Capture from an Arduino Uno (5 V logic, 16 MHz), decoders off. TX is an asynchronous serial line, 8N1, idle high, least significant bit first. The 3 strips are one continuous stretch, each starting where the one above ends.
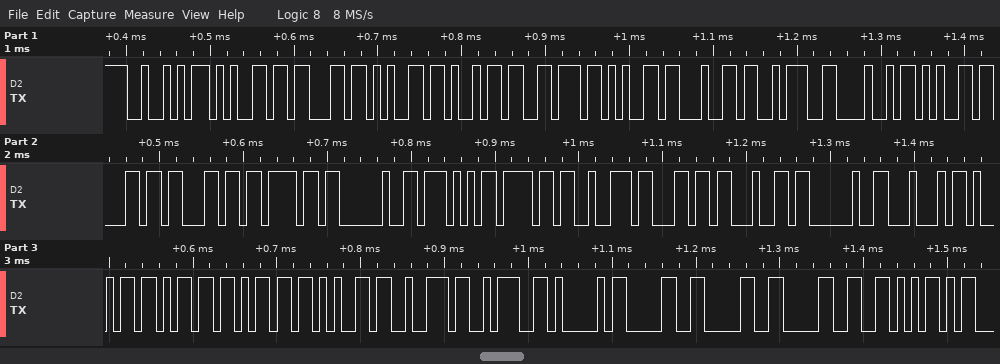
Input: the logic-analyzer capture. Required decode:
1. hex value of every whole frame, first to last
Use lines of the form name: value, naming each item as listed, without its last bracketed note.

hex value of every whole frame, first to last: 0x52 0x65 0x63 0x65 0x69 0x76 0x65 0x64 0x3A 0x48 0x65 0x6C 0x6C 0x6F 0x20 0x57 0x6F 0x72 0x6C 0x64 0x20 0x44 0x69 0x6D 0x6D 0x65 0x72 0x3A 0x41 0x30 0x30 0x30 0x56
